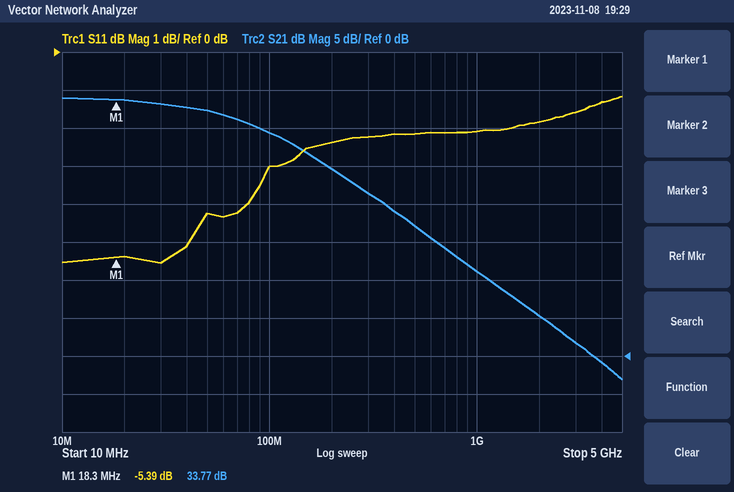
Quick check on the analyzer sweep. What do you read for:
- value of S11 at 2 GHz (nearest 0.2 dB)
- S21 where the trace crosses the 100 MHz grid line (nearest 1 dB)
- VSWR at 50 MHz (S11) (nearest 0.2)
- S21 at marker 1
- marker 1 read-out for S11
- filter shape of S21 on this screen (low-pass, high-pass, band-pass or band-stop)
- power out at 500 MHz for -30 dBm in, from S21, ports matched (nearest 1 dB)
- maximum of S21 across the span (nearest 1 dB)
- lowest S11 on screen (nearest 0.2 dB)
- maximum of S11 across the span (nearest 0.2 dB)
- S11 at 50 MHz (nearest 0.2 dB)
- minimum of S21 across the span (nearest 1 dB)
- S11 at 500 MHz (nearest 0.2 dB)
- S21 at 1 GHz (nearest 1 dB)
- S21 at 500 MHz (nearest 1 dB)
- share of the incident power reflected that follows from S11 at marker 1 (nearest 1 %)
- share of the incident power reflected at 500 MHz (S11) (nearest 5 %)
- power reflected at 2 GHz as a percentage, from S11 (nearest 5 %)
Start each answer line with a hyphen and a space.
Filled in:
- -1.8 dB
- 29 dB
- 4.2
- 33.77 dB
- -5.39 dB
- low-pass
- -13 dBm
- 34 dB
- -5.6 dB
- -1.2 dB
- -4.2 dB
- -3 dB
- -2.2 dB
- 11 dB
- 17 dB
- 29 %
- 60 %
- 65 %
